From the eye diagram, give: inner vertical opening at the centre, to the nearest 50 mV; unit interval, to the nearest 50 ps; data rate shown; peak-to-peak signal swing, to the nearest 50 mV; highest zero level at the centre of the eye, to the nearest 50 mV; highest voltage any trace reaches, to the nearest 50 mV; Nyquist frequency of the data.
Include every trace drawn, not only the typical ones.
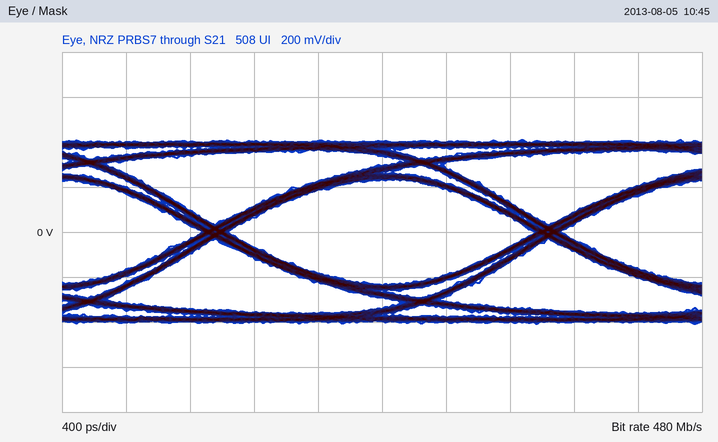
450 mV
2.10 ns
480 Mb/s
800 mV
-250 mV
400 mV
240 MHz
